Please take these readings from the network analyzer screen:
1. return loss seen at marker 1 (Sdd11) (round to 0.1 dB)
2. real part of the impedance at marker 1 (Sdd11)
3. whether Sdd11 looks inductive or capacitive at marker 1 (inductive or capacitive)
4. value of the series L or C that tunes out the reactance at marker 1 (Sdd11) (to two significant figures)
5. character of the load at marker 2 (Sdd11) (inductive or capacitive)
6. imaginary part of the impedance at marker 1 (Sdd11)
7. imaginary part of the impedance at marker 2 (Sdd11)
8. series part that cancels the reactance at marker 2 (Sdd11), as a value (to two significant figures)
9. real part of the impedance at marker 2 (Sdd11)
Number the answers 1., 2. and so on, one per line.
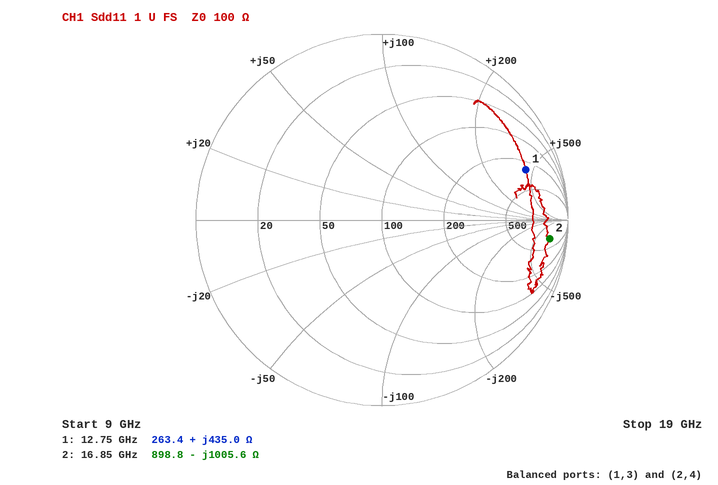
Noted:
1. 1.7 dB
2. 263.4 Ω
3. inductive
4. 29 fF
5. capacitive
6. +435.0 Ω
7. -1005.6 Ω
8. 9.5 nH
9. 898.8 Ω
